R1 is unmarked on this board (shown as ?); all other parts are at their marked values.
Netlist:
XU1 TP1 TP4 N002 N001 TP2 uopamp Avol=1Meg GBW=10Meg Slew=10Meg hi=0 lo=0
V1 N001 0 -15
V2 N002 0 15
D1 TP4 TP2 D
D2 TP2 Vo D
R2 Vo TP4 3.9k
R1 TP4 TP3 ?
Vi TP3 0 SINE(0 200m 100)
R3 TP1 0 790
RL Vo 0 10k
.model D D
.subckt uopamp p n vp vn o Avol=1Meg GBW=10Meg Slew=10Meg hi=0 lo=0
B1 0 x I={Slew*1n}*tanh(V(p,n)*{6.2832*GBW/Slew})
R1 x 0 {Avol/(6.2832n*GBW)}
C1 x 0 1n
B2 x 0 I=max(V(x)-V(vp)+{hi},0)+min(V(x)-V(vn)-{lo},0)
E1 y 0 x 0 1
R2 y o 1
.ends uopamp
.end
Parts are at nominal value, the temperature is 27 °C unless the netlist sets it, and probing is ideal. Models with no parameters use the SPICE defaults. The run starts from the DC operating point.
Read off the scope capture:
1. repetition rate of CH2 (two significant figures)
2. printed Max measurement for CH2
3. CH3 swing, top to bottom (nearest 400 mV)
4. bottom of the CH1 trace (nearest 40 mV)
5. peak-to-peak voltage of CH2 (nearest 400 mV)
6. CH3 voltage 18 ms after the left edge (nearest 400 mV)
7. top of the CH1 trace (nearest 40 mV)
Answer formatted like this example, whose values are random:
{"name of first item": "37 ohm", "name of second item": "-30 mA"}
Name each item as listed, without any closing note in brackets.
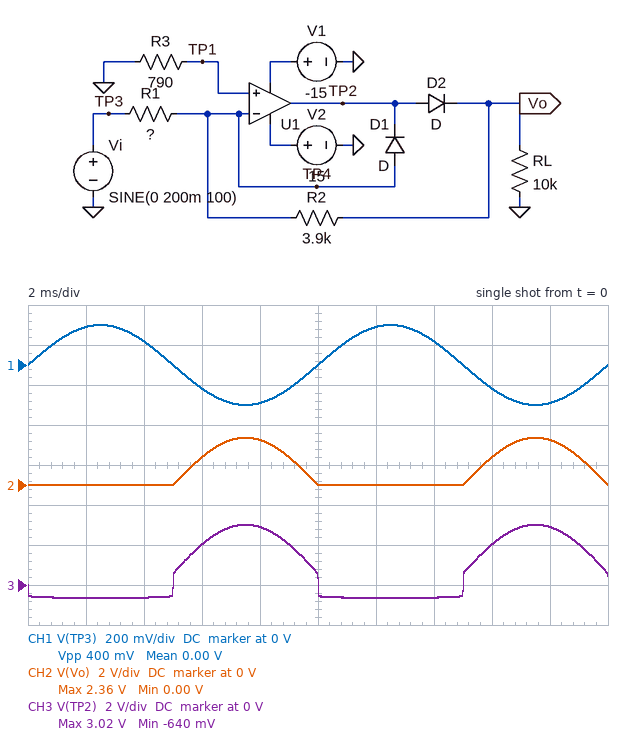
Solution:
{"repetition rate of CH2": "100 Hz", "printed Max measurement for CH2": "2.36 V", "CH3 swing, top to bottom": "3.6 V", "bottom of the CH1 trace": "-200 mV", "peak-to-peak voltage of CH2": "2.4 V", "CH3 voltage 18 ms after the left edge": "2.8 V", "top of the CH1 trace": "200 mV"}
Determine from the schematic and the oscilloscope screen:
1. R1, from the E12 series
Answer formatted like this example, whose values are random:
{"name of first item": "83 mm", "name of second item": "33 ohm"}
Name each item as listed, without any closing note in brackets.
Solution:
{"R1, from the E12 series": "330 Ω"}
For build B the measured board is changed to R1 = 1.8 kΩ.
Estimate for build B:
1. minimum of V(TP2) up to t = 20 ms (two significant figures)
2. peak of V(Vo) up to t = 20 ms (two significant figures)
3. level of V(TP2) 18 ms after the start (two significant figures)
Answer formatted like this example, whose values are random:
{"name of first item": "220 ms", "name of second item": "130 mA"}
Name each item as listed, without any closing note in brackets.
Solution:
{"minimum of V(TP2) up to t = 20 ms": "-600 mV", "peak of V(Vo) up to t = 20 ms": "430 mV", "level of V(TP2) 18 ms after the start": "1.0 V"}
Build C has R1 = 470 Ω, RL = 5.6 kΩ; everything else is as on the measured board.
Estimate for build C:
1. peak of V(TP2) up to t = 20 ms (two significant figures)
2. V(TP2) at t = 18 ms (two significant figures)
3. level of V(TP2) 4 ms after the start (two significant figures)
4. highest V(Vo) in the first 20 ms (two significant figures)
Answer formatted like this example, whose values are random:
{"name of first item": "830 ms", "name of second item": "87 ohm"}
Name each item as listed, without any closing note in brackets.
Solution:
{"peak of V(TP2) up to t = 20 ms": "2.3 V", "V(TP2) at t = 18 ms": "2.2 V", "level of V(TP2) 4 ms after the start": "-620 mV", "highest V(Vo) in the first 20 ms": "1.7 V"}
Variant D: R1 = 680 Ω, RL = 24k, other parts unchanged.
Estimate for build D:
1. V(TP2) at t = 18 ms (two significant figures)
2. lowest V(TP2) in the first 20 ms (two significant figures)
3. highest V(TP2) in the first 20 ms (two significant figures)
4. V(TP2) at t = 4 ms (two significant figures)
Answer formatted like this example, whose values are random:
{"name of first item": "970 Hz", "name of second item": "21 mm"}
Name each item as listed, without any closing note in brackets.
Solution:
{"V(TP2) at t = 18 ms": "1.7 V", "lowest V(TP2) in the first 20 ms": "-620 mV", "highest V(TP2) in the first 20 ms": "1.8 V", "V(TP2) at t = 4 ms": "-610 mV"}
